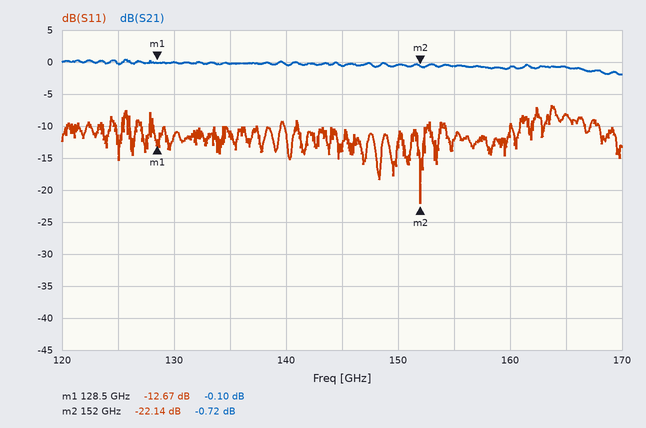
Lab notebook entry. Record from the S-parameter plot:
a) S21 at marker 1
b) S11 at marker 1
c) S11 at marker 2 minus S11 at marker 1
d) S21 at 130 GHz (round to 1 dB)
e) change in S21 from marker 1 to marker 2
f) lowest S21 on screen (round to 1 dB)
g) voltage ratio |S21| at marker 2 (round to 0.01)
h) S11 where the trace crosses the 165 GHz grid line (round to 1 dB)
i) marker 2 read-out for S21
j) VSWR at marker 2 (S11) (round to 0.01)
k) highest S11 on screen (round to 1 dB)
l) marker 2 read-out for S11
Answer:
-0.10 dB
-12.67 dB
-9.47 dB
0 dB
-0.62 dB
-2 dB
0.92
-8 dB
-0.72 dB
1.17
-7 dB
-22.14 dB
